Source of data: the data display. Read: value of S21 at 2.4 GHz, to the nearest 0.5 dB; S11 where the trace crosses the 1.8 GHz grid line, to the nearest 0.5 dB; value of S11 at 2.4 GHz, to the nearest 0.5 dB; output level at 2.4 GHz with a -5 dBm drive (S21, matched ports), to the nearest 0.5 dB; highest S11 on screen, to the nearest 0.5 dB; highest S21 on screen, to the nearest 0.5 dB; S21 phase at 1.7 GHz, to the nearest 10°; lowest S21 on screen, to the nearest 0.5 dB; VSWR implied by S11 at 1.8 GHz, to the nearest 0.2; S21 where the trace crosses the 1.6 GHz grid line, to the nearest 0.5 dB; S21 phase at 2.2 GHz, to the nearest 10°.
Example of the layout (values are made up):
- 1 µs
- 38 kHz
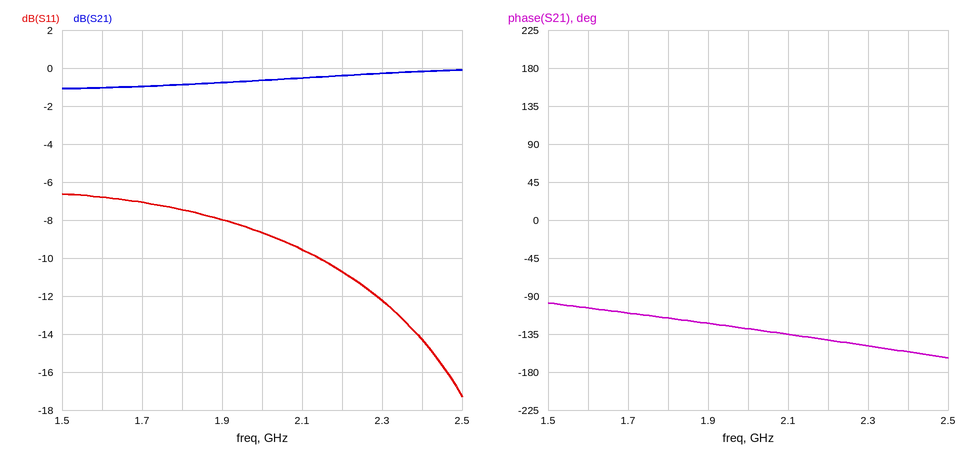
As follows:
- 0.0 dB
- -7.5 dB
- -14.5 dB
- -5.0 dBm
- -6.5 dB
- 0.0 dB
- -110°
- -1.0 dB
- 2.4
- -1.0 dB
- -140°
